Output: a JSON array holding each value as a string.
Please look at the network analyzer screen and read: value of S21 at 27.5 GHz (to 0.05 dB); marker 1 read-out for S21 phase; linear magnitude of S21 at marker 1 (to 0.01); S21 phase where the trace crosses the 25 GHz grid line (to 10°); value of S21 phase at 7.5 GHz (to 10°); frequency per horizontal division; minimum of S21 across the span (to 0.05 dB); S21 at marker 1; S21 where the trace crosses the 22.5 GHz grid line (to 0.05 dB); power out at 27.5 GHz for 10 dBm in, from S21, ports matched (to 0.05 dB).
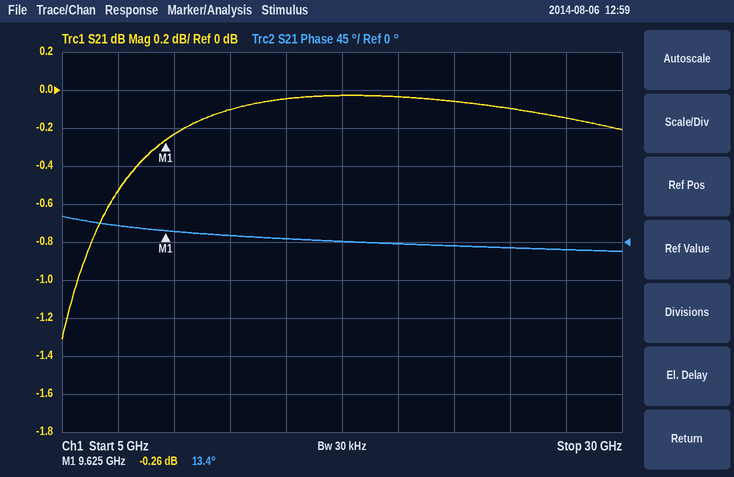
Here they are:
["-0.15 dB", "13.4°", "0.97", "-10°", "20°", "2.5 GHz", "-1.30 dB", "-0.26 dB", "-0.05 dB", "9.85 dBm"]
